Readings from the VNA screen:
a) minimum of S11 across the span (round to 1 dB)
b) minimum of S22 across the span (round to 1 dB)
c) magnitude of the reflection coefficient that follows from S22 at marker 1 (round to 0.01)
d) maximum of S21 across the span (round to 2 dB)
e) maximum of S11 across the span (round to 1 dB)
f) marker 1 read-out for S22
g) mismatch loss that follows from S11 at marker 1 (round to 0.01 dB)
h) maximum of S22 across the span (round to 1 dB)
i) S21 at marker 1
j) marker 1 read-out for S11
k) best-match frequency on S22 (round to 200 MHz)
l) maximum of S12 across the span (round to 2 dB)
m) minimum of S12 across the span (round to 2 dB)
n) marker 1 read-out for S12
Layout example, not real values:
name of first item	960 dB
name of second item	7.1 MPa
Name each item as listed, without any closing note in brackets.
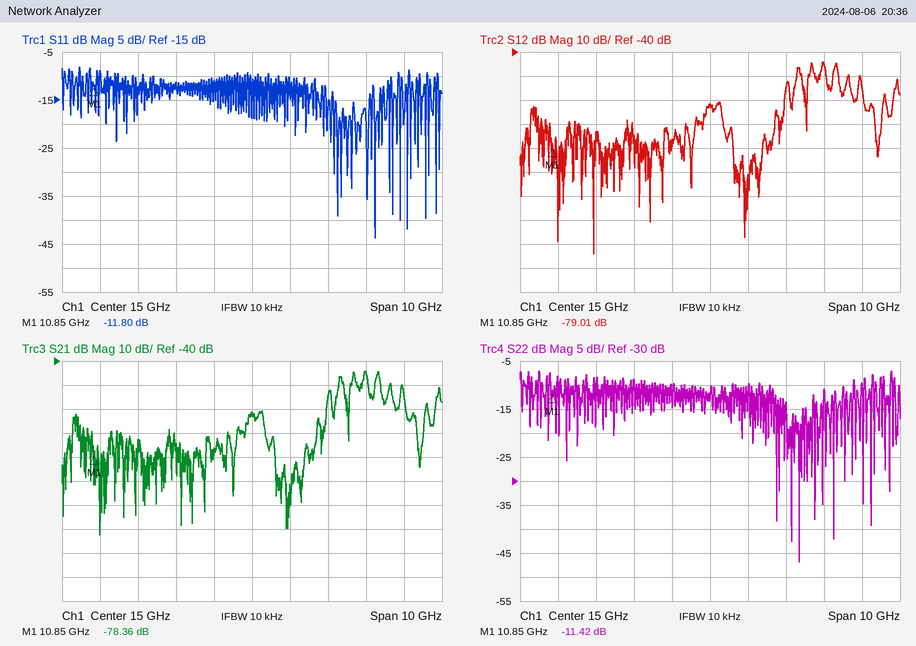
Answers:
minimum of S11 across the span	-44 dB
minimum of S22 across the span	-47 dB
magnitude of the reflection coefficient that follows from S22 at marker 1	0.27
maximum of S21 across the span	-44 dB
maximum of S11 across the span	-8 dB
marker 1 read-out for S22	-11.42 dB
mismatch loss that follows from S11 at marker 1	0.30 dB
maximum of S22 across the span	-7 dB
S21 at marker 1	-78.36 dB
marker 1 read-out for S11	-11.80 dB
best-match frequency on S22	17.4 GHz
maximum of S12 across the span	-44 dB
minimum of S12 across the span	-124 dB
marker 1 read-out for S12	-79.01 dB
